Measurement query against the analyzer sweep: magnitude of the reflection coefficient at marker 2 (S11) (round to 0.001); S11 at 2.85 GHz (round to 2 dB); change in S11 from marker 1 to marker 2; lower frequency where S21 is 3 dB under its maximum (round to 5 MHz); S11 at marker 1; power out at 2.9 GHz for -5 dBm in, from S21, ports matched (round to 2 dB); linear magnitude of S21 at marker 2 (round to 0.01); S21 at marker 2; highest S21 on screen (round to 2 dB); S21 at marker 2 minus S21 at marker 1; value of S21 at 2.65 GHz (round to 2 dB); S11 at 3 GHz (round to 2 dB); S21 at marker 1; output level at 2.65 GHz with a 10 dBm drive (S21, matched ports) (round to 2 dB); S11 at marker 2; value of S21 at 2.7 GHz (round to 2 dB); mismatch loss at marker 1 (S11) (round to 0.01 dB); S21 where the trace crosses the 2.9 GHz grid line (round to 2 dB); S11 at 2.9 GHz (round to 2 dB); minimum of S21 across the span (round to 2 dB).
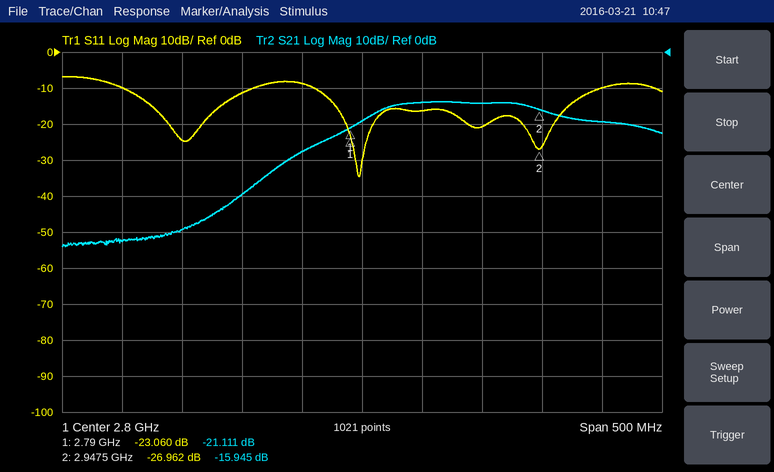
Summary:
0.045
-16 dB
-3.902 dB
2.810 GHz
-23.060 dB
-20 dBm
0.16
-15.945 dB
-14 dB
5.166 dB
-50 dB
-10 dB
-21.111 dB
-40 dBm
-26.962 dB
-40 dB
0.02 dB
-14 dB
-20 dB
-54 dB
